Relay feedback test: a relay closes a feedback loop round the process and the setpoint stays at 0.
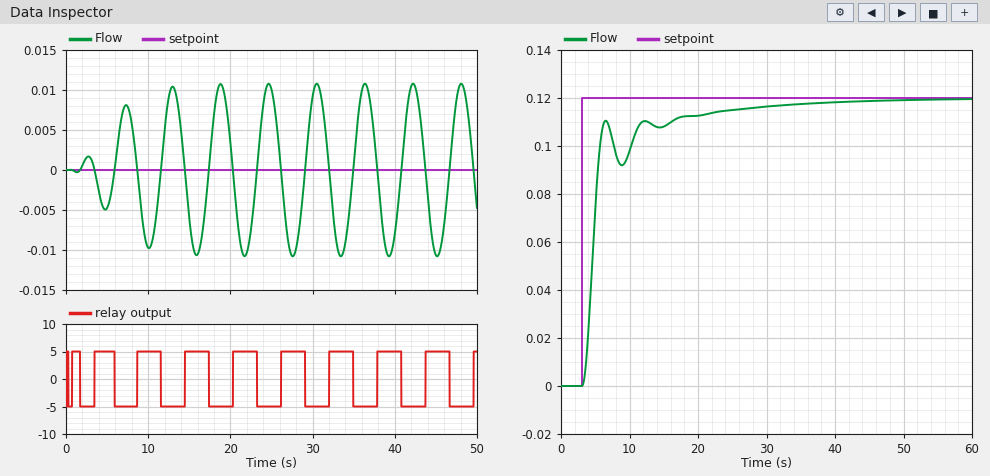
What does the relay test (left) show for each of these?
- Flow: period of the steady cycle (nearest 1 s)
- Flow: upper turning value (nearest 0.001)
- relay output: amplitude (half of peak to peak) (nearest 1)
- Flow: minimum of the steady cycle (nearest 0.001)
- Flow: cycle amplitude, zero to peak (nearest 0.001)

6 s
0.011
5
-0.011
0.011
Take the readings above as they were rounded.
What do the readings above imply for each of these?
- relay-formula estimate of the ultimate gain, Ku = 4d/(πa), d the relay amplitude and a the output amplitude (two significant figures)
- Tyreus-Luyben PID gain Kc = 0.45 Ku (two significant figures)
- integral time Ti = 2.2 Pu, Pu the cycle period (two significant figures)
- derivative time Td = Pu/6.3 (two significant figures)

580
260
13 s
0.95 s
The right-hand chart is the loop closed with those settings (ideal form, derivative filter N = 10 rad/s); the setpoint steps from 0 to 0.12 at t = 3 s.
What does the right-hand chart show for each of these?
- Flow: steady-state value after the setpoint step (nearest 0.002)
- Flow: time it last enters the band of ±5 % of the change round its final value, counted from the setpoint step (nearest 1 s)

0.120
19 s
